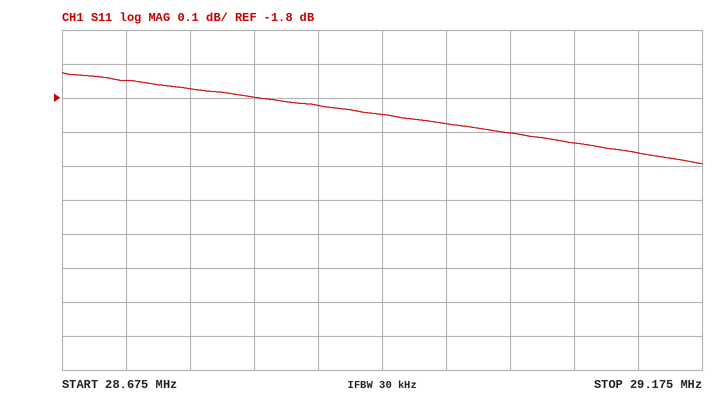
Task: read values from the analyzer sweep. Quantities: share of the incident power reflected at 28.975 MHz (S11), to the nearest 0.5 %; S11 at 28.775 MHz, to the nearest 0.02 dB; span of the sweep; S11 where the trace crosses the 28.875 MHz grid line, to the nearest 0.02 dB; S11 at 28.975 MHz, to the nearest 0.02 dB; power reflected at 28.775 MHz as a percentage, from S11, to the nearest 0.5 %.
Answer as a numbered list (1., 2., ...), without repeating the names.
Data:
1. 65.0 %
2. -1.78 dB
3. 500 kHz
4. -1.82 dB
5. -1.88 dB
6. 66.5 %
